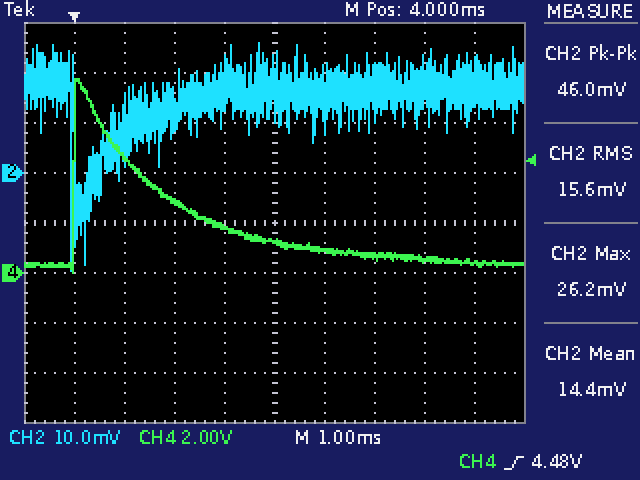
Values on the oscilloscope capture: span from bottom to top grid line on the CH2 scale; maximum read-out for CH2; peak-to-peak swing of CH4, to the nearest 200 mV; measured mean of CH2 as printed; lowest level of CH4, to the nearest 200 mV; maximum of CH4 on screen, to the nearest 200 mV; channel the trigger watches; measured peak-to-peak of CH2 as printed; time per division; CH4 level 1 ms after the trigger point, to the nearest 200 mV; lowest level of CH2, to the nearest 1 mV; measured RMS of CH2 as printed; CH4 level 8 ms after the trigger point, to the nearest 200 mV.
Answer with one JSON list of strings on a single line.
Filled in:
["80 mV", "26.2 mV", "7.8 V", "14.4 mV", "0.0 V", "7.8 V", "CH4", "46.0 mV", "1 ms", "4.6 V", "-20 mV", "15.6 mV", "400 mV"]
